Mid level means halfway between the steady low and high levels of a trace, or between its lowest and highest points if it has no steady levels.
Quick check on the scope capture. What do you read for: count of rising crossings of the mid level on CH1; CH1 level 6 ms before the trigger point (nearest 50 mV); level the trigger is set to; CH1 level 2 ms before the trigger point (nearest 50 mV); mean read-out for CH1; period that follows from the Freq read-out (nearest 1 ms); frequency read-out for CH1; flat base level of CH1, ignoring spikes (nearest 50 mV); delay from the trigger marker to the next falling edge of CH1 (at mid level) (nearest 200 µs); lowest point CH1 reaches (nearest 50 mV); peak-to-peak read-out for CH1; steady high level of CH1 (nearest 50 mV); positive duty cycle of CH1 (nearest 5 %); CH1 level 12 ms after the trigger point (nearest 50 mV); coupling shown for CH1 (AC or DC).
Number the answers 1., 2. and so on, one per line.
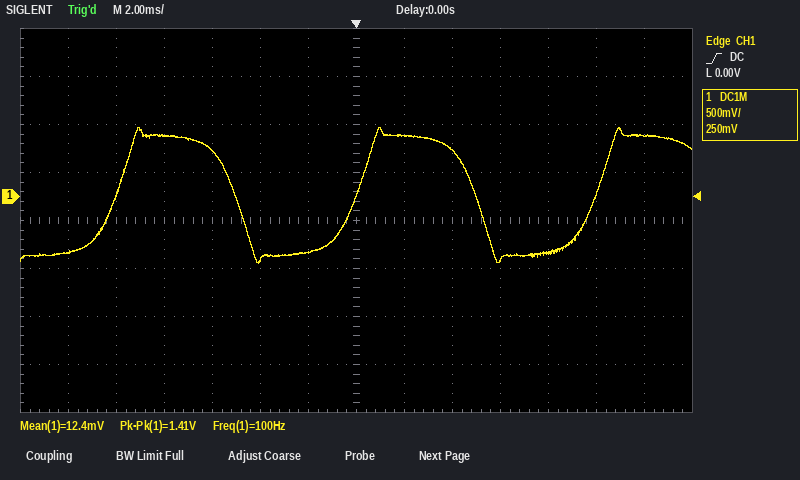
1. 3
2. 500 mV
3. 0.00 V
4. -600 mV
5. 12.4 mV
6. 10 ms
7. 100 Hz
8. -600 mV
9. 5.0 ms
10. -700 mV
11. 1.41 V
12. 650 mV
13. 50 %
14. 650 mV
15. DC
